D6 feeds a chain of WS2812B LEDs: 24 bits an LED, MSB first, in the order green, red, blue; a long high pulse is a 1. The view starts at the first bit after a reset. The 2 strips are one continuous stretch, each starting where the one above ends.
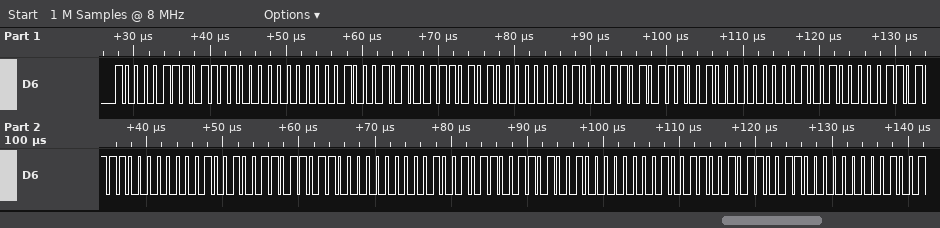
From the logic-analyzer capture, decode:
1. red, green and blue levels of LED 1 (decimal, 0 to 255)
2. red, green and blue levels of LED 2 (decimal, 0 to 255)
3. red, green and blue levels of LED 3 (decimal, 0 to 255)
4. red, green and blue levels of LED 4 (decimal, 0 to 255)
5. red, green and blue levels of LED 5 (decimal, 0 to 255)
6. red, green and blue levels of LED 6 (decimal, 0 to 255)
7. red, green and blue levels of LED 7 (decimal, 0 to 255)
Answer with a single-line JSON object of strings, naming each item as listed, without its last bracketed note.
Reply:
{"red, green and blue levels of LED 1": "120, 135, 0", "red, green and blue levels of LED 2": "117, 138, 0", "red, green and blue levels of LED 3": "114, 141, 0", "red, green and blue levels of LED 4": "111, 144, 0", "red, green and blue levels of LED 5": "108, 147, 0", "red, green and blue levels of LED 6": "105, 150, 0", "red, green and blue levels of LED 7": "102, 153, 0"}
